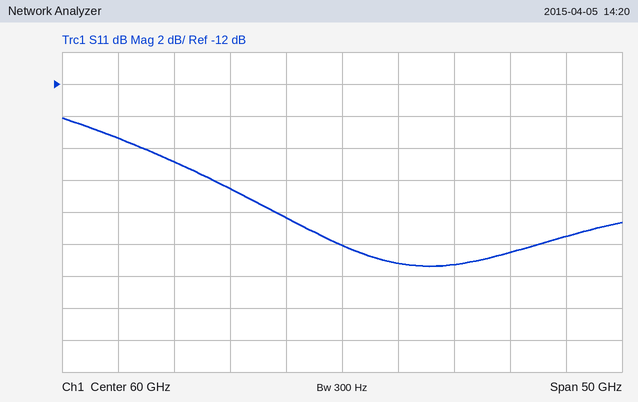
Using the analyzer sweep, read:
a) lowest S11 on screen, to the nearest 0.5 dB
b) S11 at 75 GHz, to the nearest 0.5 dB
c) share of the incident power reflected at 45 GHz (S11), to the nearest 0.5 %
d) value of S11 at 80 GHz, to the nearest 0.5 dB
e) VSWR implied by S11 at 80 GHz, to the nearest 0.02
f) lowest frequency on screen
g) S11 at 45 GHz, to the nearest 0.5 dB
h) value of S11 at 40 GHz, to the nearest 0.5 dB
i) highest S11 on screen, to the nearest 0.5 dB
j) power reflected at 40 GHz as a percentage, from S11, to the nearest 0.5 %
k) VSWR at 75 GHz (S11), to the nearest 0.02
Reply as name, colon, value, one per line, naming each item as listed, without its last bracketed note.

lowest S11 on screen, to the nearest 0.5 dB: -23.5 dB
S11 at 75 GHz, to the nearest 0.5 dB: -22.5 dB
share of the incident power reflected at 45 GHz (S11), to the nearest 0.5 %: 2.0 %
value of S11 at 80 GHz, to the nearest 0.5 dB: -21.5 dB
VSWR implied by S11 at 80 GHz, to the nearest 0.02: 1.18
lowest frequency on screen: 35 GHz
S11 at 45 GHz, to the nearest 0.5 dB: -17.0 dB
value of S11 at 40 GHz, to the nearest 0.5 dB: -15.5 dB
highest S11 on screen, to the nearest 0.5 dB: -14.0 dB
power reflected at 40 GHz as a percentage, from S11, to the nearest 0.5 %: 3.0 %
VSWR at 75 GHz (S11), to the nearest 0.02: 1.16
